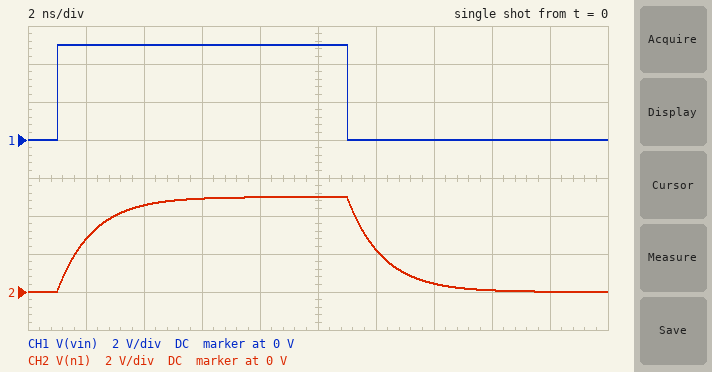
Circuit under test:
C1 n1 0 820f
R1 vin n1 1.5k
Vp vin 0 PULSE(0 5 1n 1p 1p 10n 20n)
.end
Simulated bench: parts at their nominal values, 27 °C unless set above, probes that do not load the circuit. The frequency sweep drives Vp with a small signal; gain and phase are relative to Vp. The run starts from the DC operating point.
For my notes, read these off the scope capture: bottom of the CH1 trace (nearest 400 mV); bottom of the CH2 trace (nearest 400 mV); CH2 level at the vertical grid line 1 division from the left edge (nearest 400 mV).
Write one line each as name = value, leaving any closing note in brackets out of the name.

bottom of the CH1 trace = 0 V
bottom of the CH2 trace = 0 V
CH2 level at the vertical grid line 1 division from the left edge = 2.8 V
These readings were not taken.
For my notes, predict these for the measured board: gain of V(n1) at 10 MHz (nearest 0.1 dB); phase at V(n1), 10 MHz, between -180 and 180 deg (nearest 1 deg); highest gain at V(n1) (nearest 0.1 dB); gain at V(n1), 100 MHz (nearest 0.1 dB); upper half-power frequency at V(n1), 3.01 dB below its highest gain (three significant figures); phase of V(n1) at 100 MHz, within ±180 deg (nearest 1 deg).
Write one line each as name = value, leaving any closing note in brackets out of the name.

gain of V(n1) at 10 MHz = 0 dB
phase at V(n1), 10 MHz, between -180 and 180 deg = -4 deg
highest gain at V(n1) = 0 dB
gain at V(n1), 100 MHz = -2.0 dB
upper half-power frequency at V(n1), 3.01 dB below its highest gain = 129 MHz
phase of V(n1) at 100 MHz, within ±180 deg = -38 deg
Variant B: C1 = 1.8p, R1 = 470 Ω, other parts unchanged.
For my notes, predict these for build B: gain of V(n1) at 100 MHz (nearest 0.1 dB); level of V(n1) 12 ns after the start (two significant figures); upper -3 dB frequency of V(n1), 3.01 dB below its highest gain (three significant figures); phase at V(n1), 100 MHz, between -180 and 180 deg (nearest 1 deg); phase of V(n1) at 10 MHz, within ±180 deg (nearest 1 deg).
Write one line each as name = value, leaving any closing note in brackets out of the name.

gain of V(n1) at 100 MHz = -1.1 dB
level of V(n1) 12 ns after the start = 1.5 V
upper -3 dB frequency of V(n1), 3.01 dB below its highest gain = 188 MHz
phase at V(n1), 100 MHz, between -180 and 180 deg = -28 deg
phase of V(n1) at 10 MHz, within ±180 deg = -3 deg
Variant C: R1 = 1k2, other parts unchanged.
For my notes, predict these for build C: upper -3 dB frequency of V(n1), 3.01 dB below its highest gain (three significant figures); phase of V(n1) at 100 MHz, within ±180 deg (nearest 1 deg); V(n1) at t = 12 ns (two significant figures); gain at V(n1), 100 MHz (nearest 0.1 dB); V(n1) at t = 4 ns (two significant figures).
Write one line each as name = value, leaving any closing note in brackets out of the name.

upper -3 dB frequency of V(n1), 3.01 dB below its highest gain = 162 MHz
phase of V(n1) at 100 MHz, within ±180 deg = -32 deg
V(n1) at t = 12 ns = 1.8 V
gain at V(n1), 100 MHz = -1.4 dB
V(n1) at t = 4 ns = 4.8 V
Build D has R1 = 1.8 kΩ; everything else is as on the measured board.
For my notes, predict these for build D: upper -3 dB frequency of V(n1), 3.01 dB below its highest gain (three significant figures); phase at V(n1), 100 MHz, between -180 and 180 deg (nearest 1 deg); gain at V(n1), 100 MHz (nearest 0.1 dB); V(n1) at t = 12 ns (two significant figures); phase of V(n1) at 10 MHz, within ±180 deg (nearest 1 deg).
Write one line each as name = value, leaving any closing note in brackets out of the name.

upper -3 dB frequency of V(n1), 3.01 dB below its highest gain = 108 MHz
phase at V(n1), 100 MHz, between -180 and 180 deg = -43 deg
gain at V(n1), 100 MHz = -2.7 dB
V(n1) at t = 12 ns = 2.5 V
phase of V(n1) at 10 MHz, within ±180 deg = -5 deg
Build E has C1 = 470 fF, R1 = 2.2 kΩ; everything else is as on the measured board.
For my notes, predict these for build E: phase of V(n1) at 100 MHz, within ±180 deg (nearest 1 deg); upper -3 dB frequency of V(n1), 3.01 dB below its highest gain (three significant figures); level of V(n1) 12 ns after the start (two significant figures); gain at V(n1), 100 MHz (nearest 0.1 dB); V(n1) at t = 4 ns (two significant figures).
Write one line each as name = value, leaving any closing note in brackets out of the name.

phase of V(n1) at 100 MHz, within ±180 deg = -33 deg
upper -3 dB frequency of V(n1), 3.01 dB below its highest gain = 154 MHz
level of V(n1) 12 ns after the start = 1.9 V
gain at V(n1), 100 MHz = -1.5 dB
V(n1) at t = 4 ns = 4.7 V
